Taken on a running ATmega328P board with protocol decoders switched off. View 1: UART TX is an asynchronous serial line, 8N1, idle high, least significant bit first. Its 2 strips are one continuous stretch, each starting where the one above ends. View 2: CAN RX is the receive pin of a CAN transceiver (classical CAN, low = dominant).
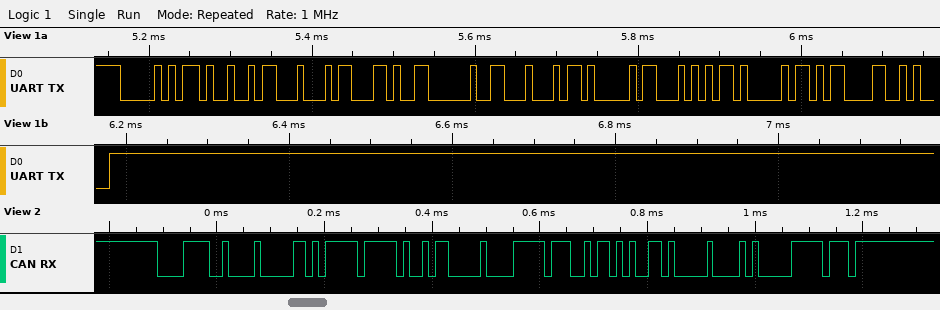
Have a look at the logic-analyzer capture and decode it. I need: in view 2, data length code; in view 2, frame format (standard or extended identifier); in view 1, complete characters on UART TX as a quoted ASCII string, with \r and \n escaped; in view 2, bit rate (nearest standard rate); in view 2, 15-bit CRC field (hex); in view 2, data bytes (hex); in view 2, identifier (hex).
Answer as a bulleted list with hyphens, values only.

- 8
- standard
- "PID, DATA\r\n"
- 83.3 kbit/s
- 0x283F
- 2B FF 96 00 FF 2D 4D 00
- 0x0F2
